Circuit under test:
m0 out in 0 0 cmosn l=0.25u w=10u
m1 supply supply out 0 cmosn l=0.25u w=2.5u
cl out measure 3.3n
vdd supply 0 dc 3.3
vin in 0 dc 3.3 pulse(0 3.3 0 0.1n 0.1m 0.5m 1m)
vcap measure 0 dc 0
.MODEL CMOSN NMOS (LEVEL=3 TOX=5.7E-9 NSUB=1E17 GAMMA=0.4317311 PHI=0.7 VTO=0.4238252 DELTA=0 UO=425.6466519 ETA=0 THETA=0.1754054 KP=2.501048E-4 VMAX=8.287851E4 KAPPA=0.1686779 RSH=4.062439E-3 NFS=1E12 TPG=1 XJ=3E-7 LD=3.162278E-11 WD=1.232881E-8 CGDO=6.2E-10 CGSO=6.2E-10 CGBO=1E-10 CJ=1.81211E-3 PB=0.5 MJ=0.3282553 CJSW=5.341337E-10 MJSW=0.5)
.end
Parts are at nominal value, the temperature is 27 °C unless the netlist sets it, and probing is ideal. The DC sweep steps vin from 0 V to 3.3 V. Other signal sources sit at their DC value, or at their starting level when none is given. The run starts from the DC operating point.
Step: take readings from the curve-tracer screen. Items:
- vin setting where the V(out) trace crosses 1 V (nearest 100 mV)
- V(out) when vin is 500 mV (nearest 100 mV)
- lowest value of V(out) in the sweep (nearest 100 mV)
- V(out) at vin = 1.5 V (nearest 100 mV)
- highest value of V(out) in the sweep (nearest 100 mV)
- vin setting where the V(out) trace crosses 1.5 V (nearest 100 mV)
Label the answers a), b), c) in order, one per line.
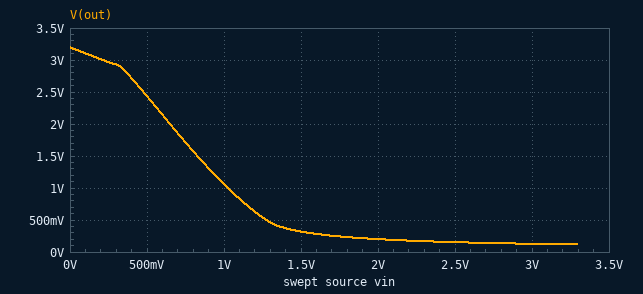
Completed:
a) 1.0 V
b) 2.4 V
c) 100 mV
d) 300 mV
e) 3.2 V
f) 800 mV
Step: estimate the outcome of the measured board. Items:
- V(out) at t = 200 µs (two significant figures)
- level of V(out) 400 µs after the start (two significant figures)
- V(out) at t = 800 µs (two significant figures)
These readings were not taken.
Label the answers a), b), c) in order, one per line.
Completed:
a) 120 mV
b) 120 mV
c) 3.0 V
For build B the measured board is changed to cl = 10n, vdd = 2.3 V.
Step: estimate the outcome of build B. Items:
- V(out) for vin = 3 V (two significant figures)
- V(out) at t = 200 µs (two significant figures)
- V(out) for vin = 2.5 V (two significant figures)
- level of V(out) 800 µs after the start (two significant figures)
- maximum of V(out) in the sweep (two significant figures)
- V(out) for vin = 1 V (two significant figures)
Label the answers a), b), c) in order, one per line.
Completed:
a) 70 mV
b) 64 mV
c) 82 mV
d) 1.9 V
e) 2.2 V
f) 310 mV
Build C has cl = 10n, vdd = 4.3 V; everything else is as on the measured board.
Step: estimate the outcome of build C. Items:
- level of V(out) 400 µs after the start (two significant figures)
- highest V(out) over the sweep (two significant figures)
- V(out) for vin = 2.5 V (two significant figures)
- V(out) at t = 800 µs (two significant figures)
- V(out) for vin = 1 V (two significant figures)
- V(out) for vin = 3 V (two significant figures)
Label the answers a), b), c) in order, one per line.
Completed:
a) 190 mV
b) 4.2 V
c) 260 mV
d) 4.0 V
e) 1.9 V
f) 210 mV
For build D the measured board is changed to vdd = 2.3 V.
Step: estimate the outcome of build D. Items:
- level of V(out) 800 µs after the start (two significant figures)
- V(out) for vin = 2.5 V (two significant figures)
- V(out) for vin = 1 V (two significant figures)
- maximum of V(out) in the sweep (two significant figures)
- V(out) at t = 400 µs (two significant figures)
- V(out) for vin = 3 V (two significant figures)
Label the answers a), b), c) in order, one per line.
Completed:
a) 2.0 V
b) 82 mV
c) 310 mV
d) 2.2 V
e) 64 mV
f) 70 mV
